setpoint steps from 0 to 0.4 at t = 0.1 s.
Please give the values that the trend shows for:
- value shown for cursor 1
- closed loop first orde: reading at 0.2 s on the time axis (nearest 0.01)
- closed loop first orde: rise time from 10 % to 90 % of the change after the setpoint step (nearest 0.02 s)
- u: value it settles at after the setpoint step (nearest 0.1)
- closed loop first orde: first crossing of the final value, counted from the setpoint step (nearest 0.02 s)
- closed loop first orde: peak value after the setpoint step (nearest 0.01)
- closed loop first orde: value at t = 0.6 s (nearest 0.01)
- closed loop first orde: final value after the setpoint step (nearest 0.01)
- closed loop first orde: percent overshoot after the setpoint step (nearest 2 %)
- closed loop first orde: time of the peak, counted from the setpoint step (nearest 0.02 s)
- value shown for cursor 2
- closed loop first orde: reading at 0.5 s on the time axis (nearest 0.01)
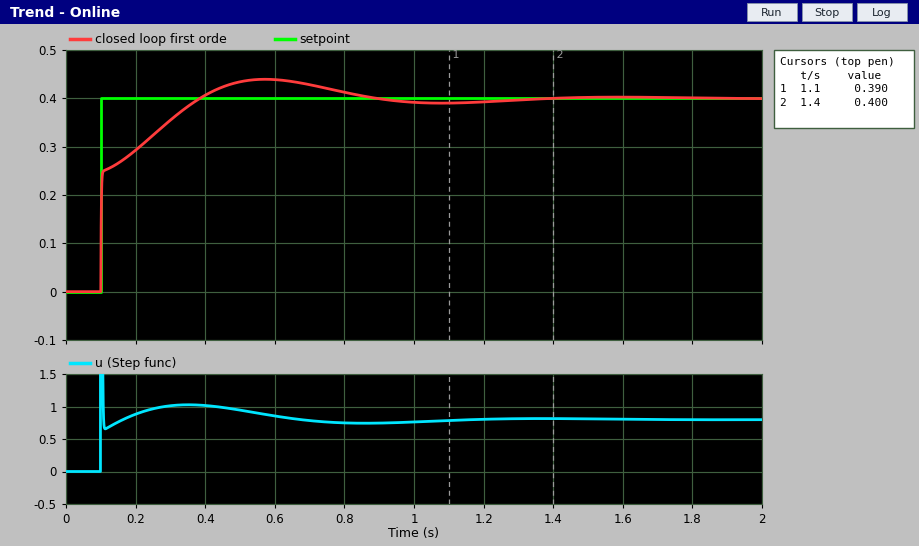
0.390
0.29
0.20 s
0.8
0.28 s
0.44
0.44
0.40
10 %
0.48 s
0.400
0.43
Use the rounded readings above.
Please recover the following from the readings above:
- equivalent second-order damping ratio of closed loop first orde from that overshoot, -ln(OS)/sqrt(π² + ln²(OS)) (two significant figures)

0.59
